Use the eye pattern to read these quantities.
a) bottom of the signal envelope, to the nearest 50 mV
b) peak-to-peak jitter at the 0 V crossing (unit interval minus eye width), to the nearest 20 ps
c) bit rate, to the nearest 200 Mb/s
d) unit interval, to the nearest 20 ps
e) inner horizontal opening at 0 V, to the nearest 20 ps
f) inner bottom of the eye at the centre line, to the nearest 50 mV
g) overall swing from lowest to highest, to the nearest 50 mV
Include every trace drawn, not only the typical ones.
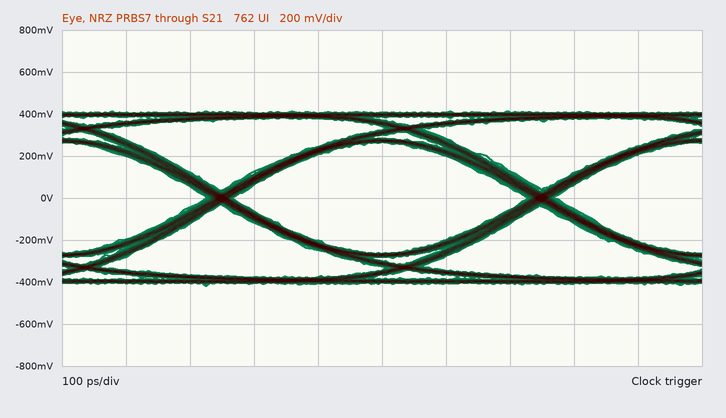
-400 mV
40 ps
2.0 Gb/s
500 ps
460 ps
-250 mV
850 mV
